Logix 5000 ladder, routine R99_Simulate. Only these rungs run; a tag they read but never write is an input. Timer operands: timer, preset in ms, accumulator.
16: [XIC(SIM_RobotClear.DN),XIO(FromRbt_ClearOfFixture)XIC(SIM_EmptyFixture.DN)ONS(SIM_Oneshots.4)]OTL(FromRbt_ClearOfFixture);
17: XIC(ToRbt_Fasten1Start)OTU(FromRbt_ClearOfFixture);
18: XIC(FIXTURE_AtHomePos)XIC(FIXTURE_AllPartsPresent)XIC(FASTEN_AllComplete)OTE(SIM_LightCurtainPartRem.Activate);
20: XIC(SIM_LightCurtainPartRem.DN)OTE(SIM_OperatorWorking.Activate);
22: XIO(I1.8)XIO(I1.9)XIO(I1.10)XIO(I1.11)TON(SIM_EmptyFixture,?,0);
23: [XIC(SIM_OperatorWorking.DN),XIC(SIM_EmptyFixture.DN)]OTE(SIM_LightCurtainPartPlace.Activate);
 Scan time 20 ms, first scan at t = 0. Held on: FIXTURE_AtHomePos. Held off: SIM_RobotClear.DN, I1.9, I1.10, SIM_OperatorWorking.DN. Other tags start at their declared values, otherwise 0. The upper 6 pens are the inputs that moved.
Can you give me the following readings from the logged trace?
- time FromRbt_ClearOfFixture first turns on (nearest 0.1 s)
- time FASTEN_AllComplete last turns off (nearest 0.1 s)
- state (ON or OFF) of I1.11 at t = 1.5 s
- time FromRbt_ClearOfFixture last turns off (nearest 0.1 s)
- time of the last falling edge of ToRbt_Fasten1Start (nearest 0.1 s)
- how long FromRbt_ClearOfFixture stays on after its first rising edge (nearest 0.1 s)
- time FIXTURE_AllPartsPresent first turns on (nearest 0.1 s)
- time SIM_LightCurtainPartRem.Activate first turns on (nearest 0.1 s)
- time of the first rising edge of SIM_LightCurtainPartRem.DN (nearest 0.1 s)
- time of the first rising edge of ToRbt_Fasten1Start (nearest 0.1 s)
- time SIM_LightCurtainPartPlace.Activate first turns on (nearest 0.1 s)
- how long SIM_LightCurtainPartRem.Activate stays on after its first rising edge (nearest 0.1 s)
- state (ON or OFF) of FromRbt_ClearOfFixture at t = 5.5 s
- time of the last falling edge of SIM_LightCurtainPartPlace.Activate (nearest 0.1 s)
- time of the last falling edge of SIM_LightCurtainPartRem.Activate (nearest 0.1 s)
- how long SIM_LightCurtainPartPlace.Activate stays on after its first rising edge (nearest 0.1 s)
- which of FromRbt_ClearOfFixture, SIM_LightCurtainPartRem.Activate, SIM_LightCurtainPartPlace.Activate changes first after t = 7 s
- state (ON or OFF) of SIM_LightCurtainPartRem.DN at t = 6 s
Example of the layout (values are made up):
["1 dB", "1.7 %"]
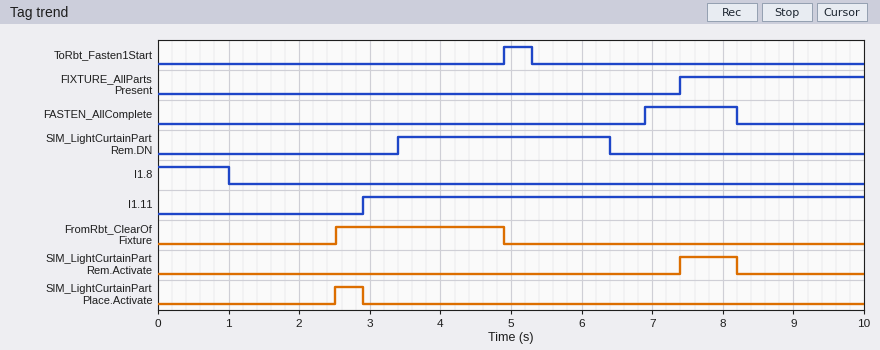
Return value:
["2.5 s", "8.2 s", "OFF", "4.9 s", "5.3 s", "2.4 s", "7.4 s", "7.4 s", "3.4 s", "4.9 s", "2.5 s", "0.8 s", "OFF", "2.9 s", "8.2 s", "0.4 s", "SIM_LightCurtainPartRem.Activate", "ON"]
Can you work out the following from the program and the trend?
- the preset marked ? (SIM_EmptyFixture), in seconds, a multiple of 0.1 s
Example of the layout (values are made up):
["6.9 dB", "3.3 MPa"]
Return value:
["1.5 s"]
